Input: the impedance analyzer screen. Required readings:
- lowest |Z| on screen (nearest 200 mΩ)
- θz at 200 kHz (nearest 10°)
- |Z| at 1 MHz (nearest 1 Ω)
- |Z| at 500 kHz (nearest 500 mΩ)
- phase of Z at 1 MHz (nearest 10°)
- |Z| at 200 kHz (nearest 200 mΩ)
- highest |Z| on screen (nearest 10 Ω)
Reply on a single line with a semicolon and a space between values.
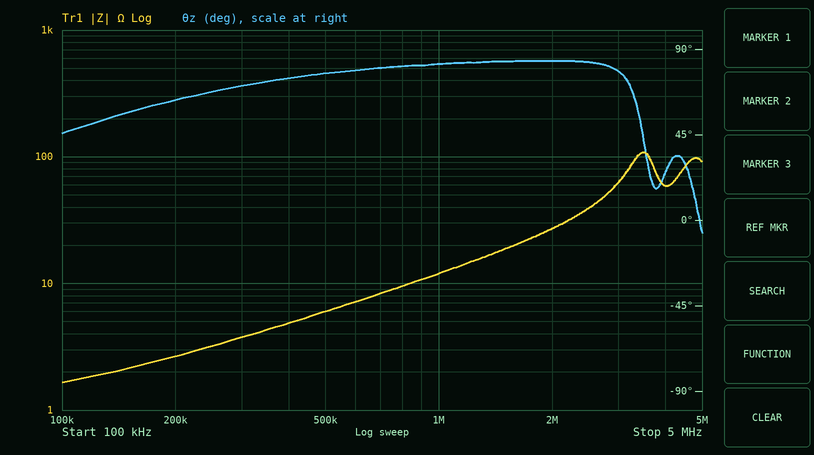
1.6 Ω; 60°; 12 Ω; 6.0 Ω; 80°; 2.6 Ω; 110 Ω
